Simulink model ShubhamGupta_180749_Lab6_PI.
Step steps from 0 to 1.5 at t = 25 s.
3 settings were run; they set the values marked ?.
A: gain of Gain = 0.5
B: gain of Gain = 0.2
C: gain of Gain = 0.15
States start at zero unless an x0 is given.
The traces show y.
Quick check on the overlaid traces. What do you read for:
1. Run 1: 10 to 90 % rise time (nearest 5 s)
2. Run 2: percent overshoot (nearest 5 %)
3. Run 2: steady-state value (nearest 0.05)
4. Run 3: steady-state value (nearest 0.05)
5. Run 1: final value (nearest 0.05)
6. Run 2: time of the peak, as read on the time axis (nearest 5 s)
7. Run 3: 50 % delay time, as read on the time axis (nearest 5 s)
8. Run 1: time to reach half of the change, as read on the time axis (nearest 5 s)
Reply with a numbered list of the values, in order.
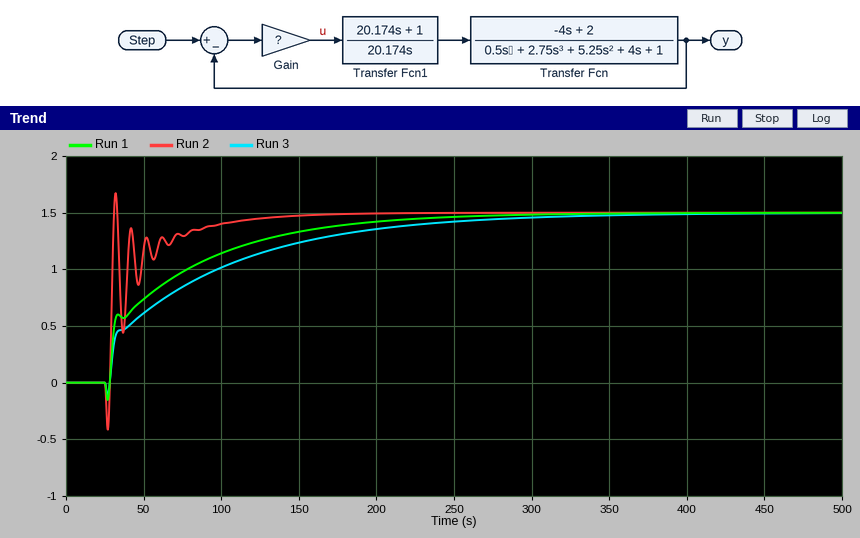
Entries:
1. 130 s
2. 10 %
3. 1.50
4. 1.50
5. 1.50
6. 30 s
7. 65 s
8. 50 s
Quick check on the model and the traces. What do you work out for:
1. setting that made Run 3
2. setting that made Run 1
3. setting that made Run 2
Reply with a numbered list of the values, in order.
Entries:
1. C
2. B
3. A
